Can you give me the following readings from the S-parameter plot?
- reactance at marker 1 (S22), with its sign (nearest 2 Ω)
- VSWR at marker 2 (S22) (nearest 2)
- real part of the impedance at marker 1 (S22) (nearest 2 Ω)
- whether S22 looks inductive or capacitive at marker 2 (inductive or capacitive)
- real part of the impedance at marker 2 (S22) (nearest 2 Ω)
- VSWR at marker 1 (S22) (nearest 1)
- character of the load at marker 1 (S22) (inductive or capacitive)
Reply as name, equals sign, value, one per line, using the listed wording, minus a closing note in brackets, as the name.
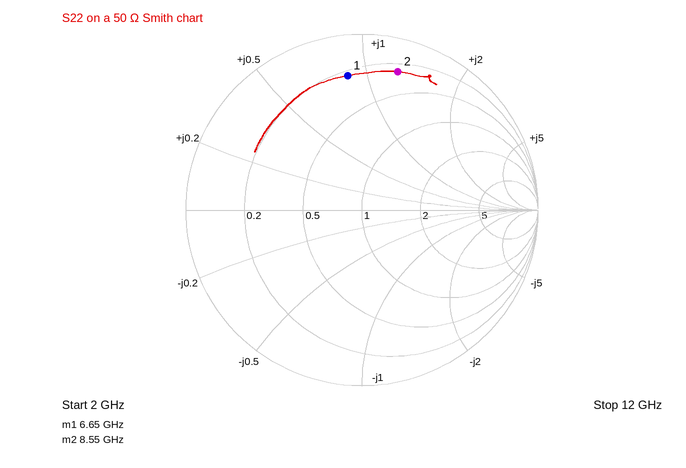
reactance at marker 1 (S22), with its sign = +44 Ω
VSWR at marker 2 (S22) = 10
real part of the impedance at marker 1 (S22) = 12 Ω
whether S22 looks inductive or capacitive at marker 2 = inductive
real part of the impedance at marker 2 (S22) = 14 Ω
VSWR at marker 1 (S22) = 8
character of the load at marker 1 (S22) = inductive
